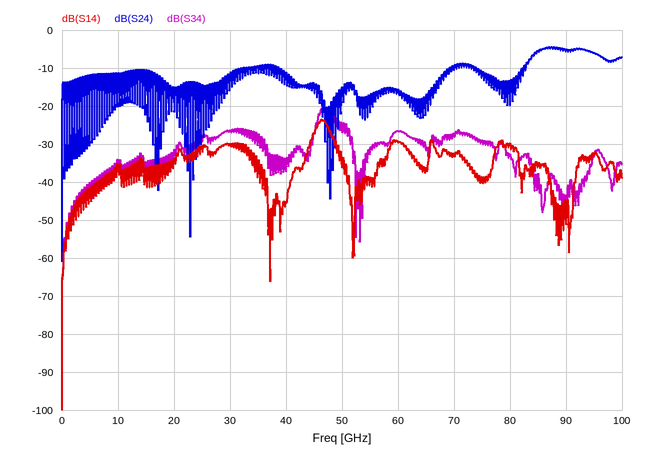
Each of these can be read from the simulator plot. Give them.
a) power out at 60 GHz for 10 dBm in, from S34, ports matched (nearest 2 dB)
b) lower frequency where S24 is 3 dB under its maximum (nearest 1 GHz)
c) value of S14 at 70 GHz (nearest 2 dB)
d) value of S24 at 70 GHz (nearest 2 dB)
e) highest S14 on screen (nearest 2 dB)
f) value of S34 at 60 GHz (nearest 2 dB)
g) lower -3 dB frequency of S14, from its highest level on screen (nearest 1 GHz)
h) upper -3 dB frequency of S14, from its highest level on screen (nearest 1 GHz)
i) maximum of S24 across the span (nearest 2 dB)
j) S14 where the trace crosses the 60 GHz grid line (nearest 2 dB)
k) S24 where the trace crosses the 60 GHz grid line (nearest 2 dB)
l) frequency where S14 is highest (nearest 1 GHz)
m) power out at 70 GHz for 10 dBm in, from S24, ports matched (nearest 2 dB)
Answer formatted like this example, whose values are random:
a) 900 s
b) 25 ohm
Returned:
a) -16 dBm
b) 84 GHz
c) -32 dB
d) -10 dB
e) -24 dB
f) -26 dB
g) 45 GHz
h) 48 GHz
i) -4 dB
j) -30 dB
k) -16 dB
l) 46 GHz
m) 0 dBm
